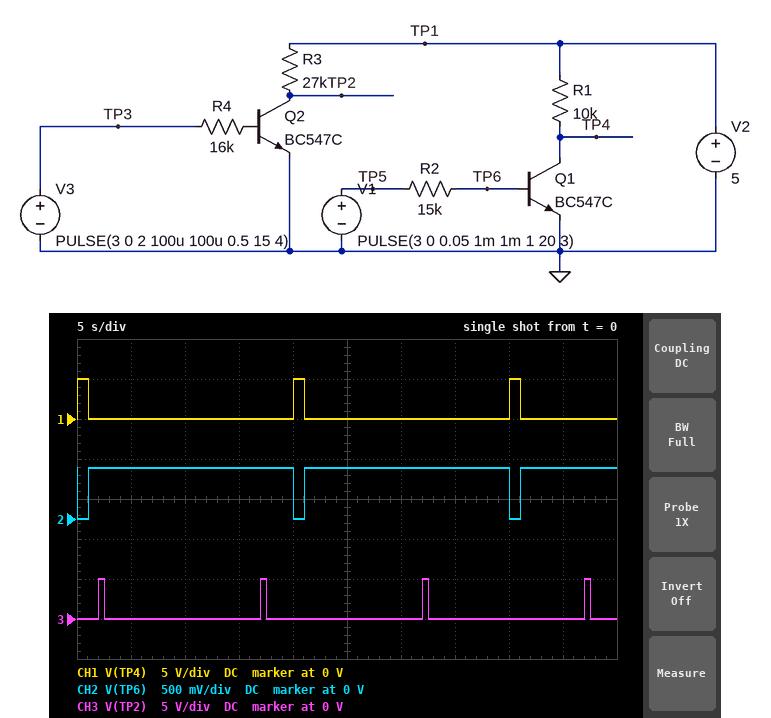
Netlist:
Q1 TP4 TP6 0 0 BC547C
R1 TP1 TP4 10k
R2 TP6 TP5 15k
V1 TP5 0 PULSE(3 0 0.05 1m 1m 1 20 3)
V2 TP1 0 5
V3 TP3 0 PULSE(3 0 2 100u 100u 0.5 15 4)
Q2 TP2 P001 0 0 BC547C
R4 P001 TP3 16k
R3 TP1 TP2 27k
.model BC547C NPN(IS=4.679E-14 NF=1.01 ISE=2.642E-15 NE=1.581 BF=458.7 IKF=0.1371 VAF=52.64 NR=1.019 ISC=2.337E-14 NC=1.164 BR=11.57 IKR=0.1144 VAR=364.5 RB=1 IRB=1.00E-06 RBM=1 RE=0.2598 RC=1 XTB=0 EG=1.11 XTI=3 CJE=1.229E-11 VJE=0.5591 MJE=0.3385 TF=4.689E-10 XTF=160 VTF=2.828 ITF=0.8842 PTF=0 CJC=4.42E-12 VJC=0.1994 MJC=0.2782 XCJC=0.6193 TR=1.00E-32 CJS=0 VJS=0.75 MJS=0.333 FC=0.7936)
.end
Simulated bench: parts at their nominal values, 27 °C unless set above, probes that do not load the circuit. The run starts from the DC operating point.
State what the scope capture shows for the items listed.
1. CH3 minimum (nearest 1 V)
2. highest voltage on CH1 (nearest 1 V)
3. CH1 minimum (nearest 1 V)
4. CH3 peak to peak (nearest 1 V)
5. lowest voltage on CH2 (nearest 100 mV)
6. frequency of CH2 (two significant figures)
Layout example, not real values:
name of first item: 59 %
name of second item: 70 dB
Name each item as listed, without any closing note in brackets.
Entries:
CH3 minimum: 0 V
highest voltage on CH1: 5 V
CH1 minimum: 0 V
CH3 peak to peak: 5 V
lowest voltage on CH2: 0 V
frequency of CH2: 50 mHz
